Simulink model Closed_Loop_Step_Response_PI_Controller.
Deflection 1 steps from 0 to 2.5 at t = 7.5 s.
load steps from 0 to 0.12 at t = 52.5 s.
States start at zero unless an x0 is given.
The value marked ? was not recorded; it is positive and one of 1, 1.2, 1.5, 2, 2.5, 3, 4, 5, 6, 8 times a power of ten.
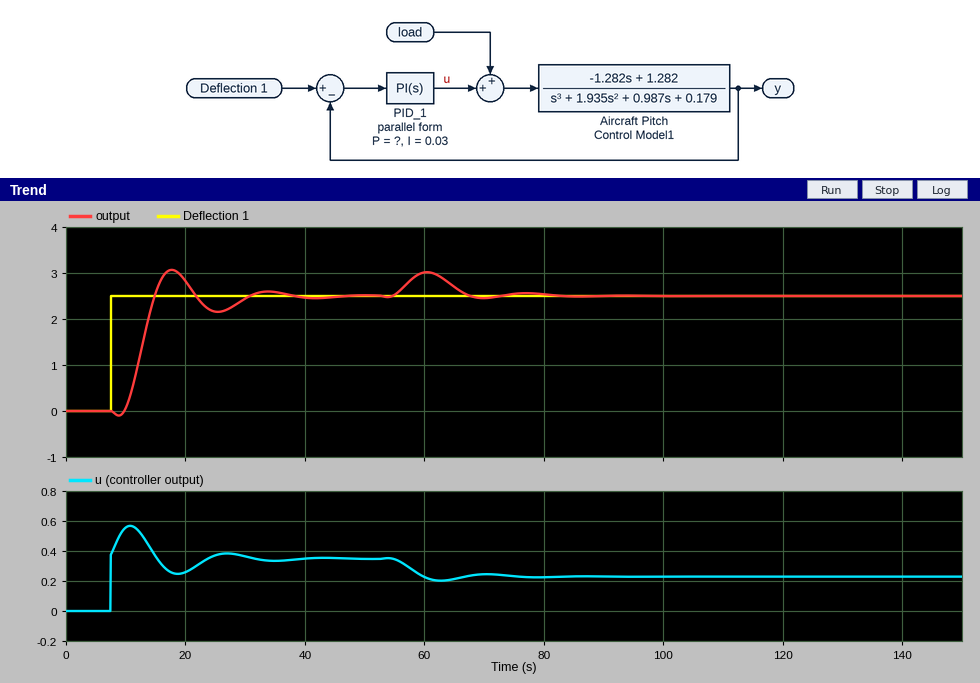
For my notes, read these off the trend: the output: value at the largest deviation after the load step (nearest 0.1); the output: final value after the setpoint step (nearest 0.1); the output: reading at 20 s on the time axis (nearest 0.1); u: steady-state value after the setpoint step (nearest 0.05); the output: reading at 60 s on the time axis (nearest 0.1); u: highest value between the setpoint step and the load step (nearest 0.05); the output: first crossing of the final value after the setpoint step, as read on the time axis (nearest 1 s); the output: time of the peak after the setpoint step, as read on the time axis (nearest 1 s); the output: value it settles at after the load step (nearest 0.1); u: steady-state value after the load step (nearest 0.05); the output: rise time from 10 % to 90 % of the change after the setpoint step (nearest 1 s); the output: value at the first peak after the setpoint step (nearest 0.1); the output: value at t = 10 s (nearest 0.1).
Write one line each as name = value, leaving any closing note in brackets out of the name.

the output: value at the largest deviation after the load step = 3.0
the output: final value after the setpoint step = 2.5
the output: reading at 20 s on the time axis = 2.8
u: steady-state value after the setpoint step = 0.35
the output: reading at 60 s on the time axis = 3.0
u: highest value between the setpoint step and the load step = 0.55
the output: first crossing of the final value after the setpoint step, as read on the time axis = 15 s
the output: time of the peak after the setpoint step, as read on the time axis = 18 s
the output: value it settles at after the load step = 2.5
u: steady-state value after the load step = 0.25
the output: rise time from 10 % to 90 % of the change after the setpoint step = 4 s
the output: value at the first peak after the setpoint step = 3.1
the output: value at t = 10 s = 0.1
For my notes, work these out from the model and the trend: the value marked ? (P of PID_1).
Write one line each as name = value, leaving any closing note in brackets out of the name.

the value marked ? = 0.15
